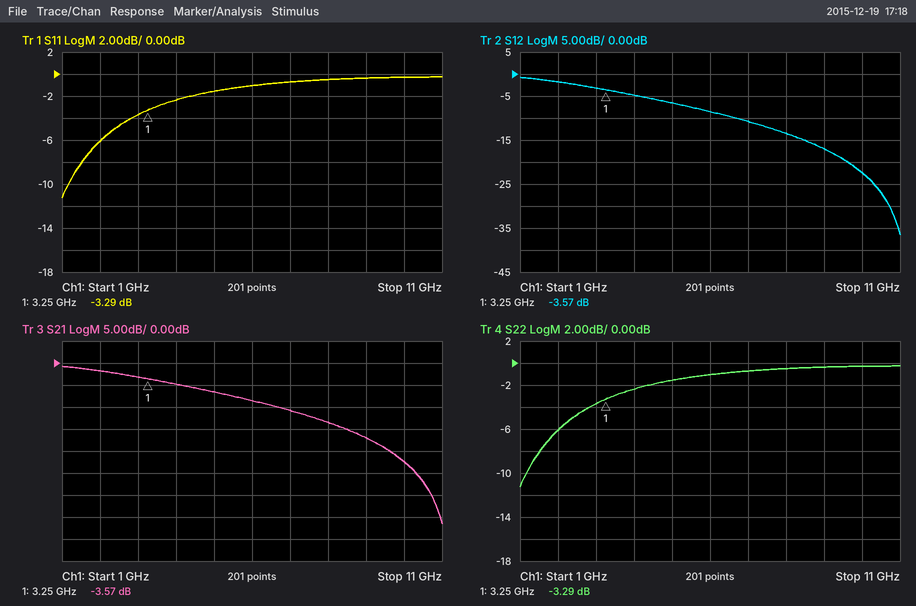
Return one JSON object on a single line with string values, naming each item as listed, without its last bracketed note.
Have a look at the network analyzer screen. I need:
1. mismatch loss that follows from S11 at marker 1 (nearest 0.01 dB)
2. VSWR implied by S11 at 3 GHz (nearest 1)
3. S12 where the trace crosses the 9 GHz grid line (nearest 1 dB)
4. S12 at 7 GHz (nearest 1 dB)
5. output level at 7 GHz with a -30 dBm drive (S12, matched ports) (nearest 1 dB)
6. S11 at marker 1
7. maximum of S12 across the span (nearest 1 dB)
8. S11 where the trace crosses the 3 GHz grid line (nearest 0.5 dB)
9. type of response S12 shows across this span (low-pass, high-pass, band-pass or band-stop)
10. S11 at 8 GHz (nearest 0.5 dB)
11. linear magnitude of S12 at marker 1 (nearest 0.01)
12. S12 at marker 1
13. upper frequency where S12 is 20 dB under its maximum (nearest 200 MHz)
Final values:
{"mismatch loss that follows from S11 at marker 1": "2.75 dB", "VSWR implied by S11 at 3 GHz": "5", "S12 where the trace crosses the 9 GHz grid line": "-17 dB", "S12 at 7 GHz": "-11 dB", "output level at 7 GHz with a -30 dBm drive (S12, matched ports)": "-41 dBm", "S11 at marker 1": "-3.29 dB", "maximum of S12 across the span": "-1 dB", "S11 where the trace crosses the 3 GHz grid line": "-3.5 dB", "type of response S12 shows across this span": "low-pass", "S11 at 8 GHz": "-0.5 dB", "linear magnitude of S12 at marker 1": "0.66", "S12 at marker 1": "-3.57 dB", "upper frequency where S12 is 20 dB under its maximum": "9.8 GHz"}
